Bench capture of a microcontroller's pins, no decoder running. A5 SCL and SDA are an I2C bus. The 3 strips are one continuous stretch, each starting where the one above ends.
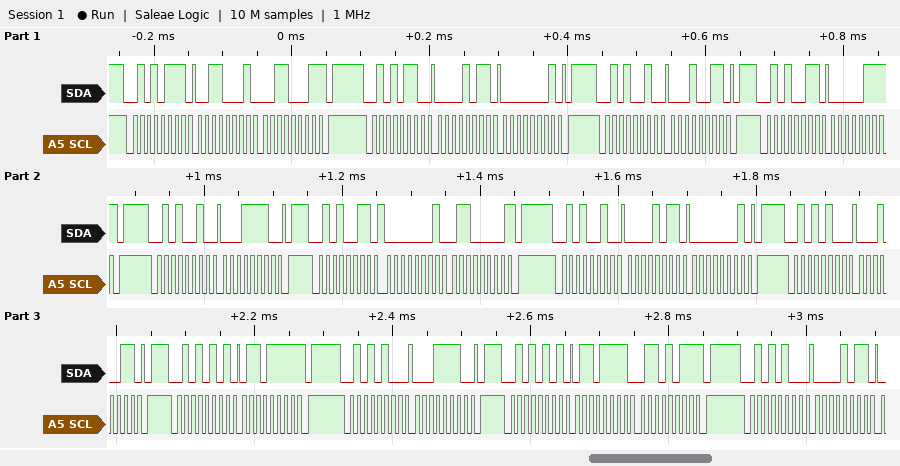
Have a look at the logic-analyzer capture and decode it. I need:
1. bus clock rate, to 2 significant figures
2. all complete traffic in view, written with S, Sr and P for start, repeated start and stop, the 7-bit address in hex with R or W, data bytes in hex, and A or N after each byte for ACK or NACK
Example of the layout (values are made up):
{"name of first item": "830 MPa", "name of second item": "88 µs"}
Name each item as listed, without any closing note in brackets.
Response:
{"bus clock rate, to 2 significant figures": "100 kHz", "all complete traffic in view, written with S, Sr and P for start, repeated start and stop, the 7-bit address in hex with R or W, data bytes in hex, and A or N after each byte for ACK or NACK": "S 2BR A 31 A 31 N P S 2BW A 0B A 01 A P S 29W A 13 A P S 29R A 07 N P S 29W A 1E A P S 29R A 01 A 60 N P S 29W A 0B A 01 A P S 2AW A 13 A P S 2AR A 6F N P S 2AW A 1E A P S 2AR A 6F A 6B N P S 2AW A 0B A"}
